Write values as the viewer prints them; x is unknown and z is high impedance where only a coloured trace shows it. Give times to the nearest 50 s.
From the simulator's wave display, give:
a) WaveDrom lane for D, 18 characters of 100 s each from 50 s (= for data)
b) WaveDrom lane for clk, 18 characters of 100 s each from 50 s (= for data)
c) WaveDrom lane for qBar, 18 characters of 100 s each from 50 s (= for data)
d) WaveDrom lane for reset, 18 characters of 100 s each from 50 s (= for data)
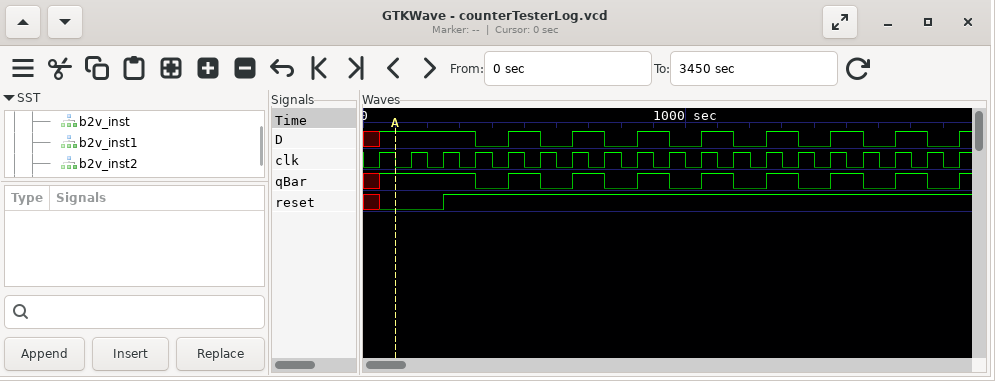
{name: 'D', wave: '1..010101010101010'}
{name: 'clk', wave: 'p.................'}
{name: 'qBar', wave: '1..010101010101010'}
{name: 'reset', wave: '0.1...............'}
